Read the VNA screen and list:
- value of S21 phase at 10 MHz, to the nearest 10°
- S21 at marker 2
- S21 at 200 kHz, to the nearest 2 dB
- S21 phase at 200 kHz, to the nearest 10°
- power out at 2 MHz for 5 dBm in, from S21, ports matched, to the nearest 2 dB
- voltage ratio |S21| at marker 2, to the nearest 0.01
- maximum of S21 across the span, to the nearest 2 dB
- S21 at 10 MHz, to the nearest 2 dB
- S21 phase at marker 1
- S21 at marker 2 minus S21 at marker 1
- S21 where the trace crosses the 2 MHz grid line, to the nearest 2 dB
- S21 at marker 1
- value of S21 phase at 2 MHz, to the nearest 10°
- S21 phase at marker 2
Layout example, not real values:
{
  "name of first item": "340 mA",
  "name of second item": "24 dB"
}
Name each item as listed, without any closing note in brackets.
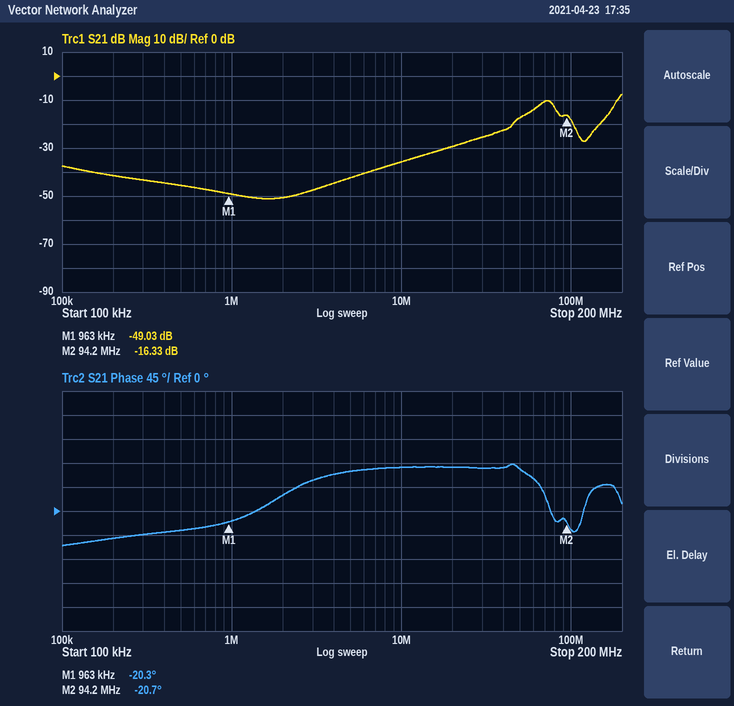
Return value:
{
  "value of S21 phase at 10 MHz, to the nearest 10°": "80°",
  "S21 at marker 2": "-16.33 dB",
  "S21 at 200 kHz, to the nearest 2 dB": "-42 dB",
  "S21 phase at 200 kHz, to the nearest 10°": "-50°",
  "power out at 2 MHz for 5 dBm in, from S21, ports matched, to the nearest 2 dB": "-46 dBm",
  "voltage ratio |S21| at marker 2, to the nearest 0.01": "0.15",
  "maximum of S21 across the span, to the nearest 2 dB": "-8 dB",
  "S21 at 10 MHz, to the nearest 2 dB": "-36 dB",
  "S21 phase at marker 1": "-20.3°",
  "S21 at marker 2 minus S21 at marker 1": "32.70 dB",
  "S21 where the trace crosses the 2 MHz grid line, to the nearest 2 dB": "-50 dB",
  "S21 at marker 1": "-49.03 dB",
  "value of S21 phase at 2 MHz, to the nearest 10°": "30°",
  "S21 phase at marker 2": "-20.7°"
}
